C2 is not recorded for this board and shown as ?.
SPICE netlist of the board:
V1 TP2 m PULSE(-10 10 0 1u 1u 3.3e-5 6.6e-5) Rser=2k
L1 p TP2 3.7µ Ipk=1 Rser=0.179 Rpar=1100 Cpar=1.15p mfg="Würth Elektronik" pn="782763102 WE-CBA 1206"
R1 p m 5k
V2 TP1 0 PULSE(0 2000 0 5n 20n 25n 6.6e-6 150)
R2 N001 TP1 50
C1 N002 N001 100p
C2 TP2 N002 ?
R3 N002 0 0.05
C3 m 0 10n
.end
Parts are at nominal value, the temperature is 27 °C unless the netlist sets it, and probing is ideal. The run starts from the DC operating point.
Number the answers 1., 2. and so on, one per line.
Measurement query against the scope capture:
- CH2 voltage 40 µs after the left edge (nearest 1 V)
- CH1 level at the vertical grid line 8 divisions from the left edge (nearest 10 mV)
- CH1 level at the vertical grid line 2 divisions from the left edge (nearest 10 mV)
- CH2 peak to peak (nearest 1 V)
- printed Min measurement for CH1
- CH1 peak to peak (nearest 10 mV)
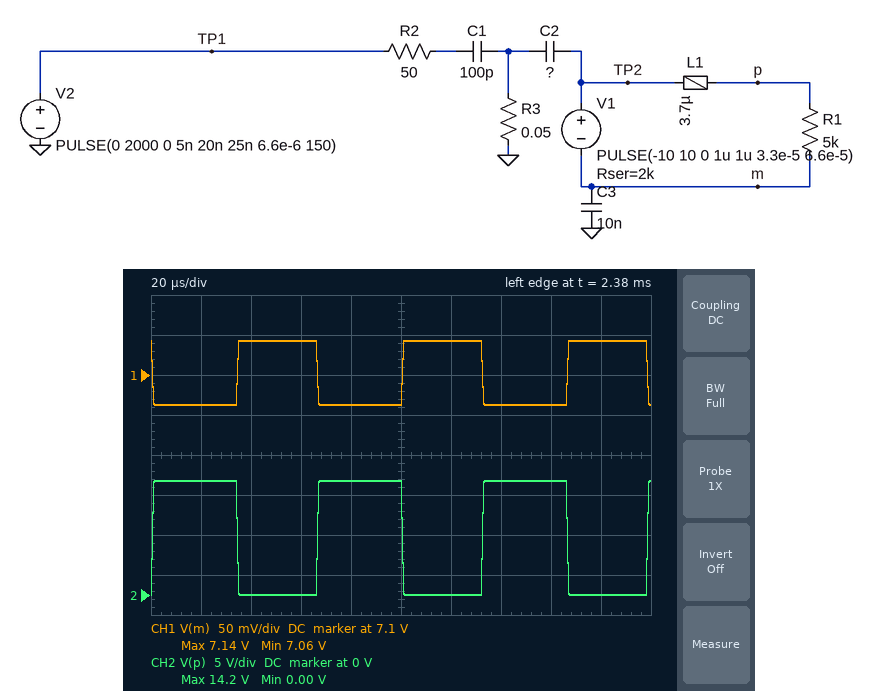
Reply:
1. 0 V
2. 7.06 V
3. 7.14 V
4. 14 V
5. 7.06 V
6. 80 mV
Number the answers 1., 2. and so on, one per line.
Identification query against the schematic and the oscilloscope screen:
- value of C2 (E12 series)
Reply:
1. 56 pF
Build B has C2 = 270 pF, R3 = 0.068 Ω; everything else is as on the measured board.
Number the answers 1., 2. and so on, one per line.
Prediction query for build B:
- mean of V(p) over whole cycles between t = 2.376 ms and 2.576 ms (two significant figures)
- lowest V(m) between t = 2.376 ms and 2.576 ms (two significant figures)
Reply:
1. 7.2 V
2. 6.8 V
